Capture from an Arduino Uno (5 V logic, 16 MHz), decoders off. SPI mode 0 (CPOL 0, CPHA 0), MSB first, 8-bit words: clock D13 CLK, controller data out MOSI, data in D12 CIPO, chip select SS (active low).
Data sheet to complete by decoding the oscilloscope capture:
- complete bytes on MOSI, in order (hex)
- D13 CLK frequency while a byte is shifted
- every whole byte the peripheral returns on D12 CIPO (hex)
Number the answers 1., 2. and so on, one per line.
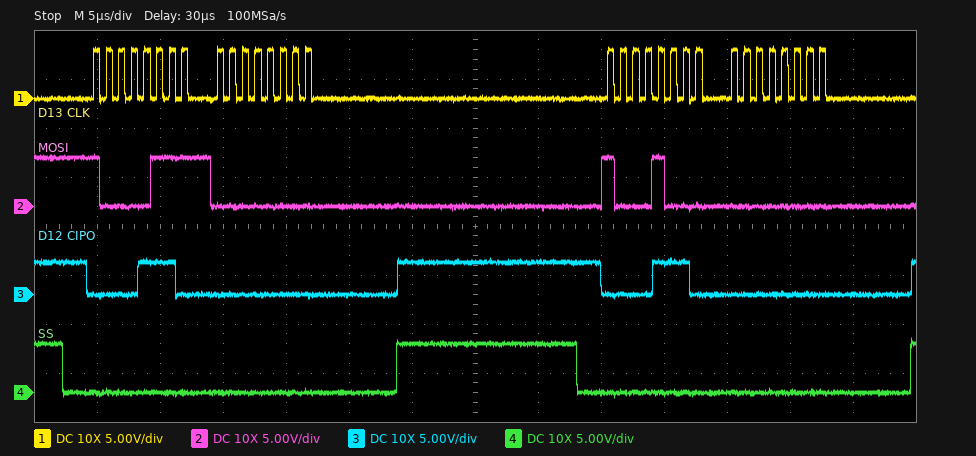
1. 87 00 88 00
2. 1 MHz
3. 0E 00 0E 00
